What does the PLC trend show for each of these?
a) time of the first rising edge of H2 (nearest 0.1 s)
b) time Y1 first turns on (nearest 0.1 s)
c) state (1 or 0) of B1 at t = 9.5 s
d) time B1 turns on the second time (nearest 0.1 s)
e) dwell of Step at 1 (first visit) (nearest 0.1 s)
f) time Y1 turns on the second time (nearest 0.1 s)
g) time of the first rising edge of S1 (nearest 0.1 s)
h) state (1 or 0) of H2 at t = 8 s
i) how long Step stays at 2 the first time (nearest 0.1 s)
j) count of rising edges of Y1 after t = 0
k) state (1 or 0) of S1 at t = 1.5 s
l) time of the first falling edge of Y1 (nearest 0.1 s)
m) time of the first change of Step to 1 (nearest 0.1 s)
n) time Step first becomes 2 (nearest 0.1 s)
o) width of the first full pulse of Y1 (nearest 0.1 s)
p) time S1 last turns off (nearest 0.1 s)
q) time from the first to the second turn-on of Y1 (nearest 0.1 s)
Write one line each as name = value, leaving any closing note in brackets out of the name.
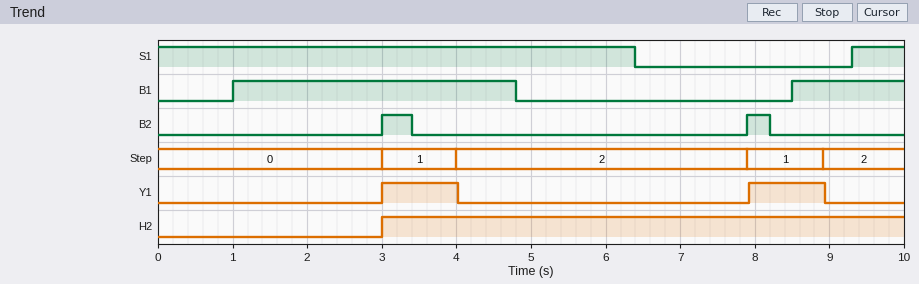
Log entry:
time of the first rising edge of H2 = 3.0 s
time Y1 first turns on = 3.0 s
state (1 or 0) of B1 at t = 9.5 s = 1
time B1 turns on the second time = 8.5 s
dwell of Step at 1 (first visit) = 1.0 s
time Y1 turns on the second time = 7.9 s
time of the first rising edge of S1 = 9.3 s
state (1 or 0) of H2 at t = 8 s = 1
how long Step stays at 2 the first time = 3.9 s
count of rising edges of Y1 after t = 0 = 2
state (1 or 0) of S1 at t = 1.5 s = 1
time of the first falling edge of Y1 = 4.0 s
time of the first change of Step to 1 = 3.0 s
time Step first becomes 2 = 4.0 s
width of the first full pulse of Y1 = 1.0 s
time S1 last turns off = 6.4 s
time from the first to the second turn-on of Y1 = 4.9 s
